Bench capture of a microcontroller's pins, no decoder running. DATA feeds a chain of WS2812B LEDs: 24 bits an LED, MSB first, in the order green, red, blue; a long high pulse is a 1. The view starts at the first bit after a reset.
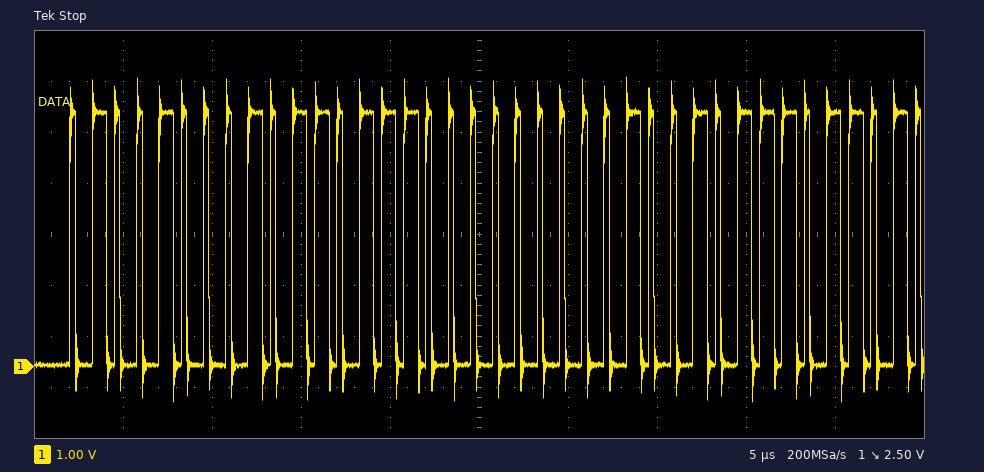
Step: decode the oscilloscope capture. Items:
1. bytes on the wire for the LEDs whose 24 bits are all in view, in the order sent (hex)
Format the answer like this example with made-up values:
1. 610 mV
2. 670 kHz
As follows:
1. 48 B7 00
